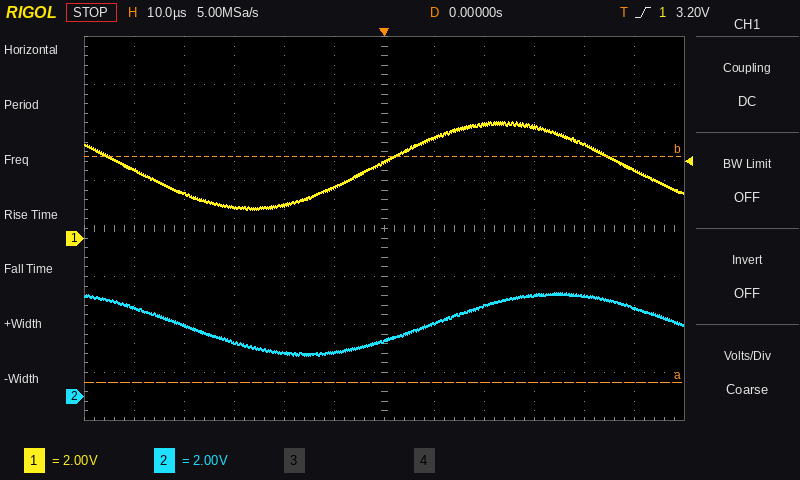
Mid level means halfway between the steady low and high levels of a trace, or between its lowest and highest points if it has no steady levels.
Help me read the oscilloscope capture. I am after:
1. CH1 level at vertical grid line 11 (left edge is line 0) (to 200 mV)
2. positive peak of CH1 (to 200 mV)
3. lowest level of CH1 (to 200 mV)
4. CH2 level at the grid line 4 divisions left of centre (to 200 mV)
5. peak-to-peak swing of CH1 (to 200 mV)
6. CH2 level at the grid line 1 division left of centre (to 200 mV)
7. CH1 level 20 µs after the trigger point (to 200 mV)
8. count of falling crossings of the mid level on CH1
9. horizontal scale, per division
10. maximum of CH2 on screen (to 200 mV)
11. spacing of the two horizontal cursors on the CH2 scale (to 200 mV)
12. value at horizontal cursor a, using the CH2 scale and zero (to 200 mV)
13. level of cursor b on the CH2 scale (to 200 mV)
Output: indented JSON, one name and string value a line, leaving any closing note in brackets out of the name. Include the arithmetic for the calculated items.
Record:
{
  "CH1 level at vertical grid line 11 (left edge is line 0)": "2.8 V",
  "positive peak of CH1": "4.8 V",
  "lowest level of CH1": "1.2 V",
  "CH2 level at the grid line 4 divisions left of centre": "3.0 V",
  "peak-to-peak swing of CH1": "4.8 V − (1.2 V) = 3.6 V",
  "CH2 level at the grid line 1 division left of centre": "1.8 V",
  "CH1 level 20 µs after the trigger point": "4.8 V",
  "count of falling crossings of the mid level on CH1": "2",
  "horizontal scale, per division": "10 µs",
  "maximum of CH2 on screen": "4.4 V",
  "spacing of the two horizontal cursors on the CH2 scale": "9.4 V",
  "value at horizontal cursor a, using the CH2 scale and zero": "600 mV",
  "level of cursor b on the CH2 scale": "10.0 V"
}
